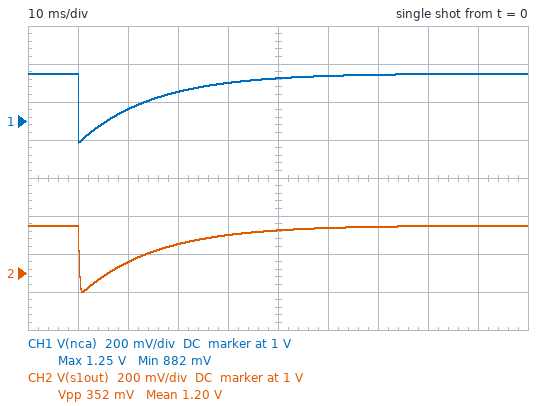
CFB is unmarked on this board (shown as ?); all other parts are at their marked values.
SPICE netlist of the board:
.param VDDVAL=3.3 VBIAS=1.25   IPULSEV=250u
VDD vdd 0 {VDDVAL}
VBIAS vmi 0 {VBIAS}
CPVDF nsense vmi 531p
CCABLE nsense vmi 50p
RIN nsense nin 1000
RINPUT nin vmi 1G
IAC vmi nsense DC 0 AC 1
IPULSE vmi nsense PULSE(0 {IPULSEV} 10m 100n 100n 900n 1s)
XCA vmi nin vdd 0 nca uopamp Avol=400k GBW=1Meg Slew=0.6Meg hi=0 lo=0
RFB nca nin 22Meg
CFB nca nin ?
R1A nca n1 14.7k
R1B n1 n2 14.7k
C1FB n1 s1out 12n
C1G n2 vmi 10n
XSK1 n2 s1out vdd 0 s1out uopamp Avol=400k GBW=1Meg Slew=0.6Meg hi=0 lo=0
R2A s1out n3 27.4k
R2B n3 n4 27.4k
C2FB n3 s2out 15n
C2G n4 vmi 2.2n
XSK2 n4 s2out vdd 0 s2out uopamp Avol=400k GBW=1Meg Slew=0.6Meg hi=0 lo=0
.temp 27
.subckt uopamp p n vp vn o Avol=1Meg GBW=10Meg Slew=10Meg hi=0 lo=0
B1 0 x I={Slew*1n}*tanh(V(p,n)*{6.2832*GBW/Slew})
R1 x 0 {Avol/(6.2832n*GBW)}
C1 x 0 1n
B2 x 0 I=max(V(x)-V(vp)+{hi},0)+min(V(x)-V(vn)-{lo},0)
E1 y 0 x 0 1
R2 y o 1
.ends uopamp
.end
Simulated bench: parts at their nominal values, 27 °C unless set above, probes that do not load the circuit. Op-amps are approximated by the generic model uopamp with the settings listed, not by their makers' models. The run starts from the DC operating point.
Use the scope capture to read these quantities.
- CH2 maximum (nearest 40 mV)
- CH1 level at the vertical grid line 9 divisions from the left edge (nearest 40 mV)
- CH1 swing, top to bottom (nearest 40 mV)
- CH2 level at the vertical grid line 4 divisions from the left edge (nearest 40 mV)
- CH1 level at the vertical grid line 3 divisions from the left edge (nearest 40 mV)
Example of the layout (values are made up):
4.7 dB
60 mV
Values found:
1.24 V
1.24 V
360 mV
1.20 V
1.16 V
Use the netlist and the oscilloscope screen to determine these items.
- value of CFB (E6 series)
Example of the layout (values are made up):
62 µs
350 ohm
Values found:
680 pF
